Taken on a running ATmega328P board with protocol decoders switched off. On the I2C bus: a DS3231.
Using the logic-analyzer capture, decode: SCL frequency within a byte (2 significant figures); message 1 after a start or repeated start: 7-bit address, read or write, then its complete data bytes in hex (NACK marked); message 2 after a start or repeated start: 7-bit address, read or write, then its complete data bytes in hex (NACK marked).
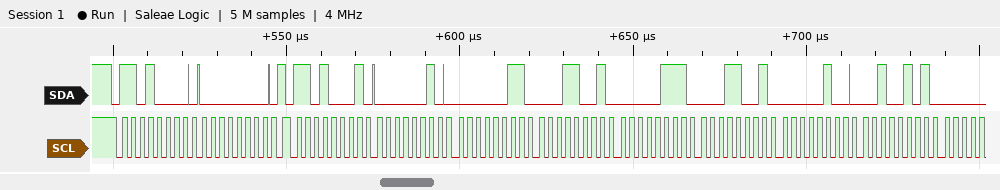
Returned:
400 kHz
0x68 write: 00
0x68 read: 02 03 19 07 19 04 25
